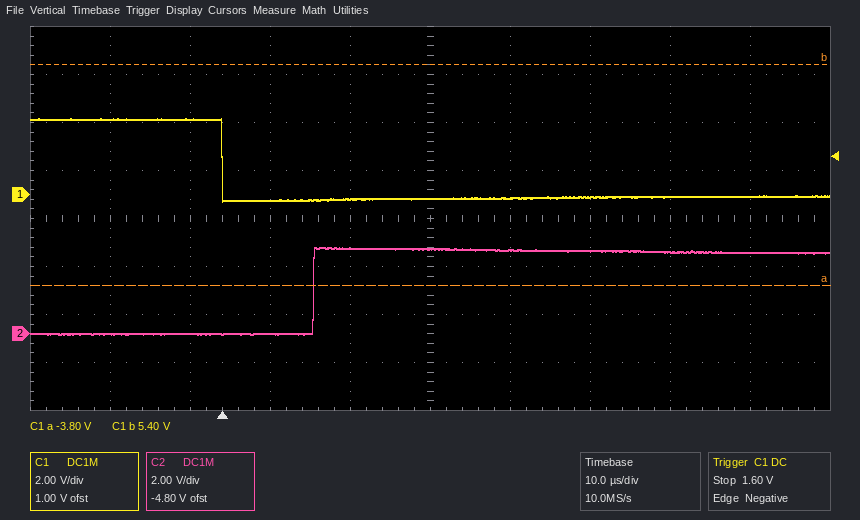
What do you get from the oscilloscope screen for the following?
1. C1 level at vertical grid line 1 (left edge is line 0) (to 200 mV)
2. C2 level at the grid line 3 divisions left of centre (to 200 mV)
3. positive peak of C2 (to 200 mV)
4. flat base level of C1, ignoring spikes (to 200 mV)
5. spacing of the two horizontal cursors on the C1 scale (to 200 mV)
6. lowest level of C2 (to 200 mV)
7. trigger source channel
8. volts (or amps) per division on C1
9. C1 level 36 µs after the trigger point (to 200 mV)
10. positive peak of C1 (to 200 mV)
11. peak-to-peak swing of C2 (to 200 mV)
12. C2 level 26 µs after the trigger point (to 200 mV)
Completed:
3.2 V
0.0 V
3.6 V
-200 mV
9.2 V
0.0 V
C1
2 V
-200 mV
3.2 V
3.6 V
3.6 V
